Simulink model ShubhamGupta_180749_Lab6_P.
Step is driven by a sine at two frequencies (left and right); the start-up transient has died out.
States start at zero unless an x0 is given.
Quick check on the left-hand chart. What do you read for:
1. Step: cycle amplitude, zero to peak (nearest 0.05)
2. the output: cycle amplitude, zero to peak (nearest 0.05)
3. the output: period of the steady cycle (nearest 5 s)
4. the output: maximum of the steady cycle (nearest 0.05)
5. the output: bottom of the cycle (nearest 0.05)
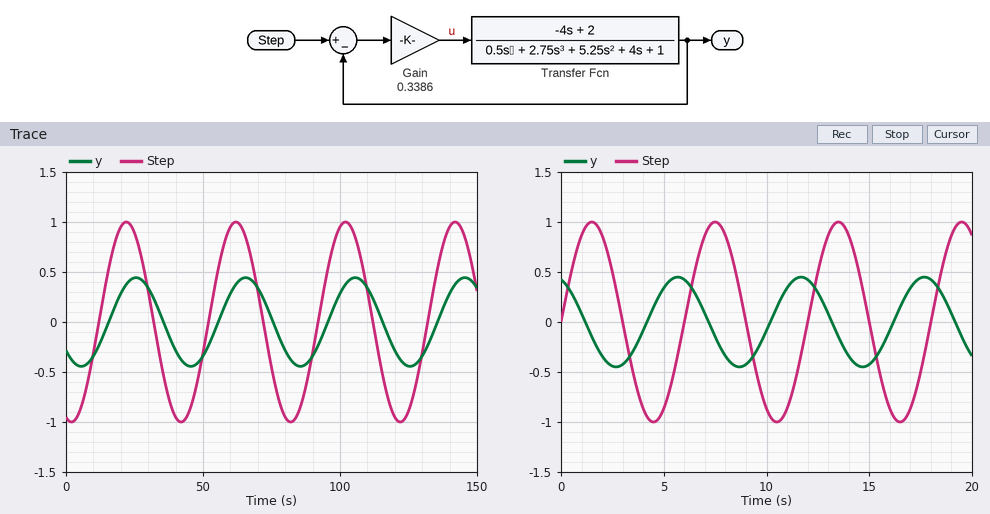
1.00
0.45
40 s
0.45
-0.45
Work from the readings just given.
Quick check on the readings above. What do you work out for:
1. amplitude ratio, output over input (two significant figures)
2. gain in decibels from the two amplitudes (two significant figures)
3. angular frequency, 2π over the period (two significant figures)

0.45
-6.9 dB
0.16 rad/s
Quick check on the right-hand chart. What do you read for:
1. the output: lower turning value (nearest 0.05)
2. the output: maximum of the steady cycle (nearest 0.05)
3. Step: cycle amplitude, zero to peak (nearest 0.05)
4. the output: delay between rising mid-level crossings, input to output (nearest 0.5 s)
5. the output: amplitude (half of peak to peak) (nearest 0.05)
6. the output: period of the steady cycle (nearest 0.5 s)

-0.45
0.45
1.00
4.0 s
0.45
6.0 s
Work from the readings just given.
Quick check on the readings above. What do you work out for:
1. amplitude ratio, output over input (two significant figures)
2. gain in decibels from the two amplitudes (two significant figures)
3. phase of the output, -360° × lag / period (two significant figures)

0.45
-6.9 dB
-240°
